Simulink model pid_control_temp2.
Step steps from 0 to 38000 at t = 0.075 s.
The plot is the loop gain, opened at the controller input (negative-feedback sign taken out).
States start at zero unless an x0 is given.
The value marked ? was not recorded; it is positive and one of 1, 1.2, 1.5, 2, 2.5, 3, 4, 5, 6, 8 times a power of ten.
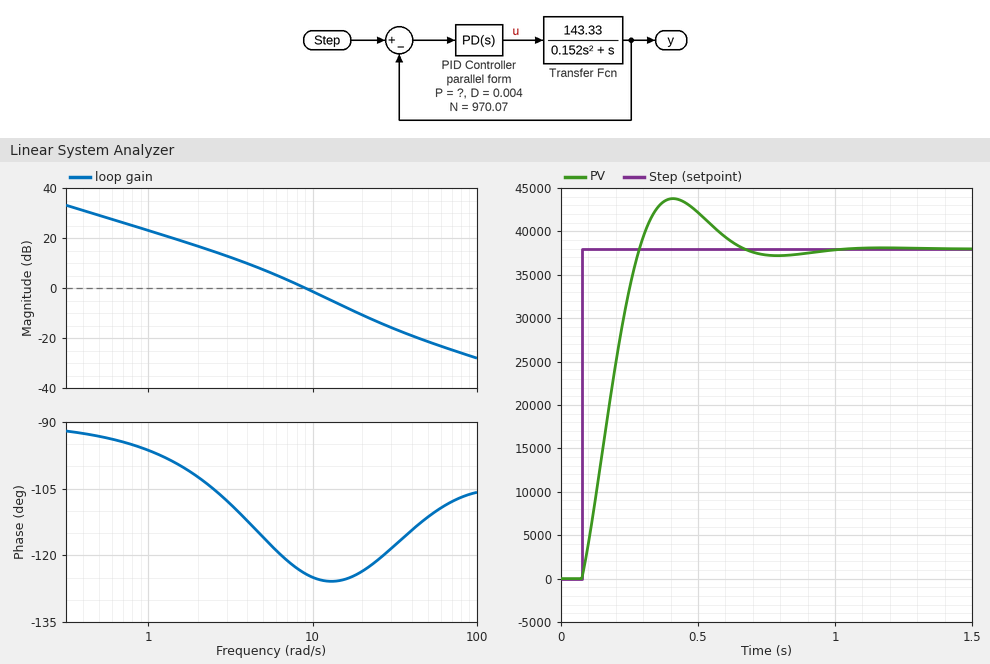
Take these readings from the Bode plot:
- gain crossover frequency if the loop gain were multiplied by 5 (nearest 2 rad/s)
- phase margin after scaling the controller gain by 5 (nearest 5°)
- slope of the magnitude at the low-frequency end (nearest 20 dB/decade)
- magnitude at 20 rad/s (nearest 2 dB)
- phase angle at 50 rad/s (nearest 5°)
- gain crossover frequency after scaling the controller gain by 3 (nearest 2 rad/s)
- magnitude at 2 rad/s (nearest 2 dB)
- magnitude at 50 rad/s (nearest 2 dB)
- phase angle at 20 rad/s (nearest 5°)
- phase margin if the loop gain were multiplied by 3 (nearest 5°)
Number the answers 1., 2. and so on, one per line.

1. 26 rad/s
2. 60°
3. -20 dB/decade
4. -10 dB
5. -110°
6. 18 rad/s
7. 16 dB
8. -22 dB
9. -125°
10. 55°
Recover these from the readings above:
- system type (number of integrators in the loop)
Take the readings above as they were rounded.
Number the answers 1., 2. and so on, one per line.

1. 1
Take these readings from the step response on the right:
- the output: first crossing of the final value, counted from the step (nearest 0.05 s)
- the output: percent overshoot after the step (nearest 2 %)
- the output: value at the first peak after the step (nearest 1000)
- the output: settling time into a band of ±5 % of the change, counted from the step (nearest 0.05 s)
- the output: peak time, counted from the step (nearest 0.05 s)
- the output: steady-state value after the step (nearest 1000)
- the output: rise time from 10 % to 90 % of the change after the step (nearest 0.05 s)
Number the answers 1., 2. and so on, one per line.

1. 0.20 s
2. 16 %
3. 44000
4. 0.50 s
5. 0.35 s
6. 38000
7. 0.15 s
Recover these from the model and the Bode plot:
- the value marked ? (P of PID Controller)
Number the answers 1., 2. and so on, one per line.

1. 0.1
